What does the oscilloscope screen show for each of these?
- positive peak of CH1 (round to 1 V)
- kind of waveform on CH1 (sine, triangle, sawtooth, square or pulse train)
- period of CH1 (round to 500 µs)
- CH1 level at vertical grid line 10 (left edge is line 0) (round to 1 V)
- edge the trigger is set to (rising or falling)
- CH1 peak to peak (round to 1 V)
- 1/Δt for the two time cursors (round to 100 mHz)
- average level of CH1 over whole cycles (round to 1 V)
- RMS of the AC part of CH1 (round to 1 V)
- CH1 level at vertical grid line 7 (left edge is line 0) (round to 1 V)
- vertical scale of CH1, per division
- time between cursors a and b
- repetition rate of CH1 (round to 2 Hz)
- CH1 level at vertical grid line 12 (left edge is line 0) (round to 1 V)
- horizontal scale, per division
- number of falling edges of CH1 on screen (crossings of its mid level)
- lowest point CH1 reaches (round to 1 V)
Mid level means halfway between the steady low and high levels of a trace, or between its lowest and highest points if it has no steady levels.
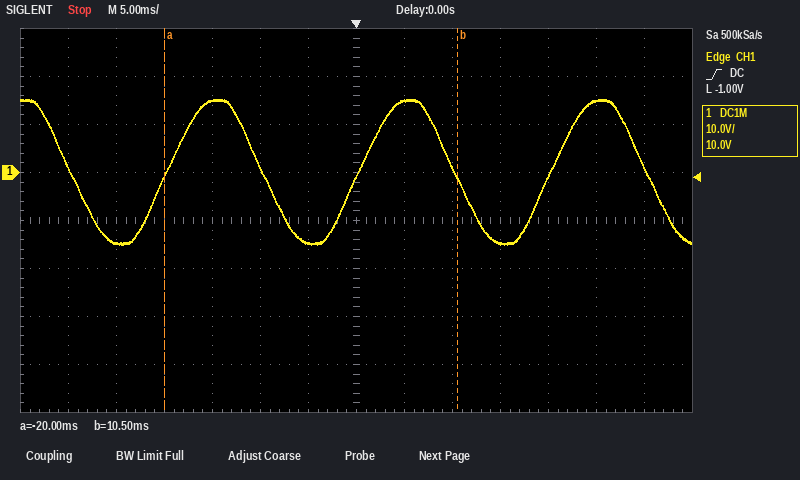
15 V
sine
20.0 ms
-15 V
rising
30 V
32.8 Hz
0 V
11 V
-1 V
10 V
30.5 ms
50 Hz
15 V
5 ms
4
-15 V
